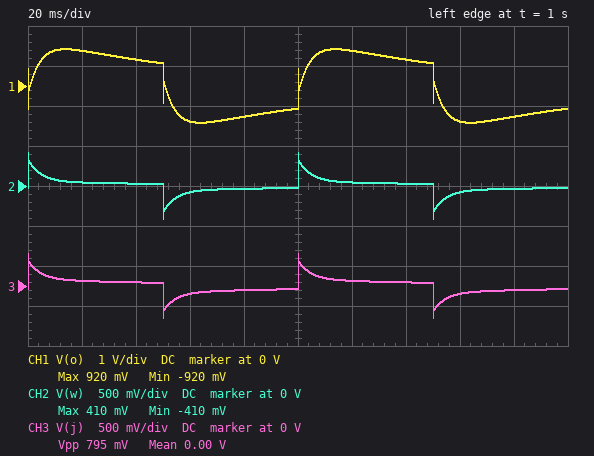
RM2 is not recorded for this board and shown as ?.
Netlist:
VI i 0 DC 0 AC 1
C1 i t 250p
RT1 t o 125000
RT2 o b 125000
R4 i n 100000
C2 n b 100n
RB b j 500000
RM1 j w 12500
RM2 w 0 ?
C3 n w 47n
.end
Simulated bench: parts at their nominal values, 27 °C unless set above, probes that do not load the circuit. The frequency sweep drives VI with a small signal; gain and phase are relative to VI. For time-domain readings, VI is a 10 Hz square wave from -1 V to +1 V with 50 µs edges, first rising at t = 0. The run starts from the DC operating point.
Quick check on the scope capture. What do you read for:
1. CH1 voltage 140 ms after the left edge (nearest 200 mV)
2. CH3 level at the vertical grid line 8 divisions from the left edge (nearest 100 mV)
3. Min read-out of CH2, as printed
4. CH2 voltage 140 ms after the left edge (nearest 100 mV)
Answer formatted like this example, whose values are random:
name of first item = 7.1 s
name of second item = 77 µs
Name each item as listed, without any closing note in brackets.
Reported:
CH1 voltage 140 ms after the left edge = 600 mV
CH3 level at the vertical grid line 8 divisions from the left edge = -100 mV
Min read-out of CH2, as printed = -410 mV
CH2 voltage 140 ms after the left edge = 0 V
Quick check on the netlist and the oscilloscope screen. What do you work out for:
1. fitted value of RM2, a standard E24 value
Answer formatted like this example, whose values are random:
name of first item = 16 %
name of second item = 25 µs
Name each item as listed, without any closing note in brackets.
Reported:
fitted value of RM2, a standard E24 value = 22 kΩ
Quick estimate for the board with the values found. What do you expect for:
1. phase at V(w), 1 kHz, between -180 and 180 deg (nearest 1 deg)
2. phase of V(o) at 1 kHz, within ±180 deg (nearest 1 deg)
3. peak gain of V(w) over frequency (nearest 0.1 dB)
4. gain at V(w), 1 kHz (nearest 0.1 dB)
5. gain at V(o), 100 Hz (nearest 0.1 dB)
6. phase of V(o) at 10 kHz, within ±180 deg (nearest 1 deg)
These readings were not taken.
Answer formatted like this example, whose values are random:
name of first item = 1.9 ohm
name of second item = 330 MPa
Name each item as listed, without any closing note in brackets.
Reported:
phase at V(w), 1 kHz, between -180 and 180 deg = 8 deg
phase of V(o) at 1 kHz, within ±180 deg = 28 deg
peak gain of V(w) over frequency = -12.6 dB
gain at V(w), 1 kHz = -14.5 dB
gain at V(o), 100 Hz = -10.0 dB
phase of V(o) at 10 kHz, within ±180 deg = 9 deg
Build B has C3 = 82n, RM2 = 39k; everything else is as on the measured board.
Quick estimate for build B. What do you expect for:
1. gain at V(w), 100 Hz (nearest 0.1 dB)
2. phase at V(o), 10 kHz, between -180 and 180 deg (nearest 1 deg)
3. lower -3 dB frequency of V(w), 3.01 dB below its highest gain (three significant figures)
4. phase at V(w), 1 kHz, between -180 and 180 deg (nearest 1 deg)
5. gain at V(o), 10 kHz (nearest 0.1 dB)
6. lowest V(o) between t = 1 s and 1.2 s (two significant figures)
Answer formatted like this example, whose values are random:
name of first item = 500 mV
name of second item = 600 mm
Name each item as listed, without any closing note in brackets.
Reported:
gain at V(w), 100 Hz = -11.2 dB
phase at V(o), 10 kHz, between -180 and 180 deg = 7 deg
lower -3 dB frequency of V(w), 3.01 dB below its highest gain = 33.4 Hz
phase at V(w), 1 kHz, between -180 and 180 deg = 6 deg
gain at V(o), 10 kHz = -3.6 dB
lowest V(o) between t = 1 s and 1.2 s = -820 mV
